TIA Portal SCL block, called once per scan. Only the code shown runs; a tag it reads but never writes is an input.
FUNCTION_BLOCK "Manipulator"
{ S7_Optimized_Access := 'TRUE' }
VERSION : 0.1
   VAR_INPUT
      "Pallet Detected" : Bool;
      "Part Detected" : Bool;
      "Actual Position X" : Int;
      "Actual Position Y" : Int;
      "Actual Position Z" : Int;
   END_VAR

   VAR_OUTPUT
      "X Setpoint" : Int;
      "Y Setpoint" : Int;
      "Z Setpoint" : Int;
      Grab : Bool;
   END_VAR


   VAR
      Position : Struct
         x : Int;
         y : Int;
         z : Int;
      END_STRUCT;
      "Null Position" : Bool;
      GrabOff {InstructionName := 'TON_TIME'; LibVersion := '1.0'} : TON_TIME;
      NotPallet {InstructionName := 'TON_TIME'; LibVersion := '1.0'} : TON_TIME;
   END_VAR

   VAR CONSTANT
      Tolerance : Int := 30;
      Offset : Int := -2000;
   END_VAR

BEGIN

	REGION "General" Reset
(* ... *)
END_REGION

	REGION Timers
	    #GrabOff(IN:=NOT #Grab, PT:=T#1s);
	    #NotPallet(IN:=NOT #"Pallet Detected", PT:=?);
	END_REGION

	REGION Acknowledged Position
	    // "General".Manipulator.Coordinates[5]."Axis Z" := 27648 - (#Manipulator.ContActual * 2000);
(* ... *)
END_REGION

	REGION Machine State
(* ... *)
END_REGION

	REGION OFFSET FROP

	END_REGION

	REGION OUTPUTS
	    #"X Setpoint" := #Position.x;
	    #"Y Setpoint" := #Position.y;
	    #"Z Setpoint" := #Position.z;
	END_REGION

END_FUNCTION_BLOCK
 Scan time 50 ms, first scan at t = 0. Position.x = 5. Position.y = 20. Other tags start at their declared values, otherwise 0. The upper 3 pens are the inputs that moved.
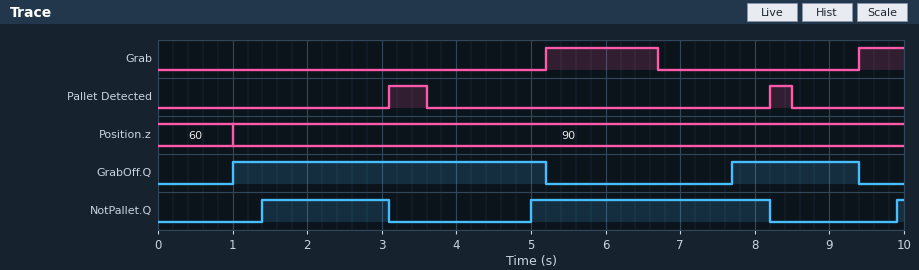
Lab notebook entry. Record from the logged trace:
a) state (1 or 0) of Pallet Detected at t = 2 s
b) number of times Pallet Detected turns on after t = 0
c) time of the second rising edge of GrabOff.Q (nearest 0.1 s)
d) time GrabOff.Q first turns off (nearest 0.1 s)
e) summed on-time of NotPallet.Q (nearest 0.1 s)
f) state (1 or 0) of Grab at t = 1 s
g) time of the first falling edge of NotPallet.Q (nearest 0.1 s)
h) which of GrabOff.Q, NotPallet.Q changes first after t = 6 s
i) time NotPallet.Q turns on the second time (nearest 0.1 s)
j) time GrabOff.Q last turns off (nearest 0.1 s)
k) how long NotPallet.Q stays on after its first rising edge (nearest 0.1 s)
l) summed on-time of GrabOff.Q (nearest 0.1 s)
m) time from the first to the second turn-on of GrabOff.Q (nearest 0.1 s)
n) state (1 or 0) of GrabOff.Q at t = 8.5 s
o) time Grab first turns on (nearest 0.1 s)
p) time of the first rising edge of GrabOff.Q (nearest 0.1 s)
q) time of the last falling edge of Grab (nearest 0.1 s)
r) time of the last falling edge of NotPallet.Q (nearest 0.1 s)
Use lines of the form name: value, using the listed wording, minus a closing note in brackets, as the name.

state (1 or 0) of Pallet Detected at t = 2 s: 0
number of times Pallet Detected turns on after t = 0: 2
time of the second rising edge of GrabOff.Q: 7.7 s
time GrabOff.Q first turns off: 5.2 s
summed on-time of NotPallet.Q: 5.0 s
state (1 or 0) of Grab at t = 1 s: 0
time of the first falling edge of NotPallet.Q: 3.1 s
which of GrabOff.Q, NotPallet.Q changes first after t = 6 s: GrabOff.Q
time NotPallet.Q turns on the second time: 5.0 s
time GrabOff.Q last turns off: 9.4 s
how long NotPallet.Q stays on after its first rising edge: 1.7 s
summed on-time of GrabOff.Q: 5.9 s
time from the first to the second turn-on of GrabOff.Q: 6.7 s
state (1 or 0) of GrabOff.Q at t = 8.5 s: 1
time Grab first turns on: 5.2 s
time of the first rising edge of GrabOff.Q: 1.0 s
time of the last falling edge of Grab: 6.7 s
time of the last falling edge of NotPallet.Q: 8.2 s
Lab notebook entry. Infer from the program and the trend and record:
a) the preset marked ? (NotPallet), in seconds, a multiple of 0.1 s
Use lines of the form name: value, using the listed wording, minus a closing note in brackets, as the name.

the preset marked ? (NotPallet), in seconds, a multiple of 0.1 s: 1.4 s
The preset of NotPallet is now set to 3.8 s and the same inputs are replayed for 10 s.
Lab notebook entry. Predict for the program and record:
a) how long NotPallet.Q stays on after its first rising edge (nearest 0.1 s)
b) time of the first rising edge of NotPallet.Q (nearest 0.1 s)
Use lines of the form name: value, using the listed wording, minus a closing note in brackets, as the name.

how long NotPallet.Q stays on after its first rising edge: 0.8 s
time of the first rising edge of NotPallet.Q: 7.4 s
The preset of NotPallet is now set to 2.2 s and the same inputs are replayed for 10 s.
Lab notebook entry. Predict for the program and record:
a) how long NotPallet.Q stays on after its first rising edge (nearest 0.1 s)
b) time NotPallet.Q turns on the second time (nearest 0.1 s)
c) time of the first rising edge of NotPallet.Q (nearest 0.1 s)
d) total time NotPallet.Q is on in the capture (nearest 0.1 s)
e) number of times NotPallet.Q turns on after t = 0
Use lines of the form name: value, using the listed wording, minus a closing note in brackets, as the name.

how long NotPallet.Q stays on after its first rising edge: 0.9 s
time NotPallet.Q turns on the second time: 5.8 s
time of the first rising edge of NotPallet.Q: 2.2 s
total time NotPallet.Q is on in the capture: 3.3 s
number of times NotPallet.Q turns on after t = 0: 2
